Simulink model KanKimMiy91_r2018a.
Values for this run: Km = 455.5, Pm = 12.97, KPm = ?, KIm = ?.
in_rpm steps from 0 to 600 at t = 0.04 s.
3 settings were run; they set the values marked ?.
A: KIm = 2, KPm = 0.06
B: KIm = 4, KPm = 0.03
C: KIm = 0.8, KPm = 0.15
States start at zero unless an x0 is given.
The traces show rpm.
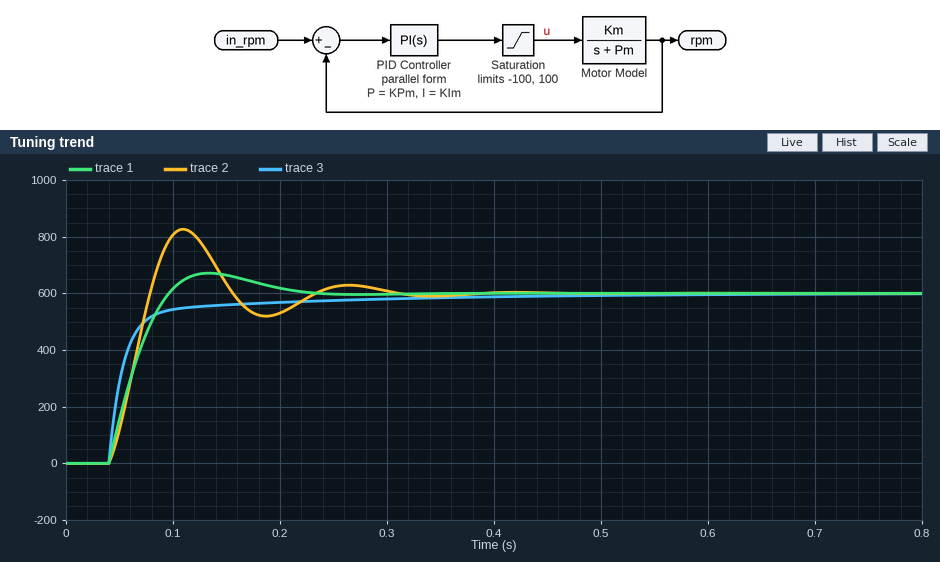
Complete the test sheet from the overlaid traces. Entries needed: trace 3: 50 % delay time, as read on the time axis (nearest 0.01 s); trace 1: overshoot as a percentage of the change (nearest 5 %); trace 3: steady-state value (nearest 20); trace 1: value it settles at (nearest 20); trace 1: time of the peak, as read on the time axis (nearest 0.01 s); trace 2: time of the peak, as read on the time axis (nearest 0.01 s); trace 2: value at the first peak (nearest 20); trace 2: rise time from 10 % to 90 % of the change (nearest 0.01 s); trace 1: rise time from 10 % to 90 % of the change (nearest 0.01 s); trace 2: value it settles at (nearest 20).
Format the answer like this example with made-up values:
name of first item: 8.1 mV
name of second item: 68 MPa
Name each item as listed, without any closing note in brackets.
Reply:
trace 3: 50 % delay time, as read on the time axis: 0.05 s
trace 1: overshoot as a percentage of the change: 10 %
trace 3: steady-state value: 600
trace 1: value it settles at: 600
trace 1: time of the peak, as read on the time axis: 0.13 s
trace 2: time of the peak, as read on the time axis: 0.11 s
trace 2: value at the first peak: 820
trace 2: rise time from 10 % to 90 % of the change: 0.03 s
trace 1: rise time from 10 % to 90 % of the change: 0.04 s
trace 2: value it settles at: 600
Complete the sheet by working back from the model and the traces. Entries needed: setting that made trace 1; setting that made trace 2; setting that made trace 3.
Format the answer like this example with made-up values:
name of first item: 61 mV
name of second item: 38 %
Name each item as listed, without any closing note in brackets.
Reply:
setting that made trace 1: A
setting that made trace 2: B
setting that made trace 3: C
